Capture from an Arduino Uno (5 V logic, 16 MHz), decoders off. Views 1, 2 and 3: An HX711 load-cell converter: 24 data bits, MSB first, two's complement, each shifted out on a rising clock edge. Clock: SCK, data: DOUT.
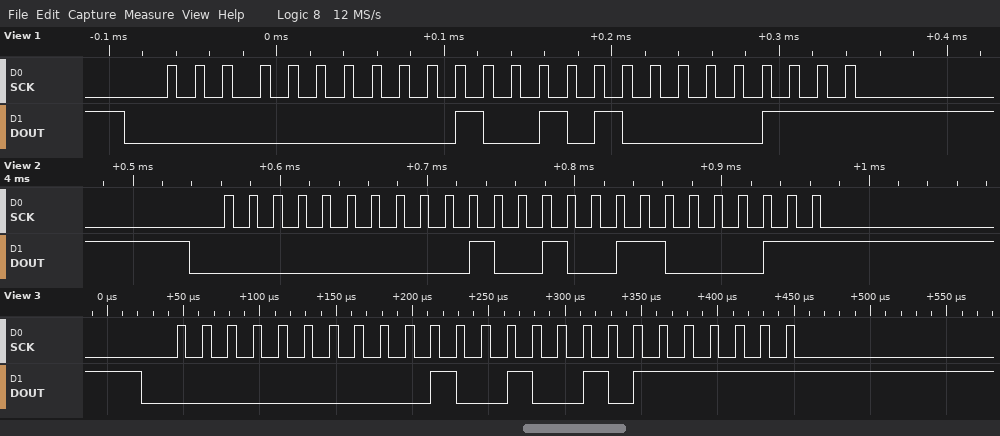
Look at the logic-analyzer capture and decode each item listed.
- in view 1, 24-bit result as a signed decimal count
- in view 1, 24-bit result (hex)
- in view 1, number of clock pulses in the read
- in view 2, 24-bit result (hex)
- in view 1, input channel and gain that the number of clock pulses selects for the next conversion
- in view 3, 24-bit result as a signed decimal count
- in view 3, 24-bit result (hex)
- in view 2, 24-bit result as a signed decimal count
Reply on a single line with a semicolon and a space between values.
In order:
9479; 0x002507; 25; 0x0024C3; channel A, gain 128; 9407; 0x0024BF; 9411
